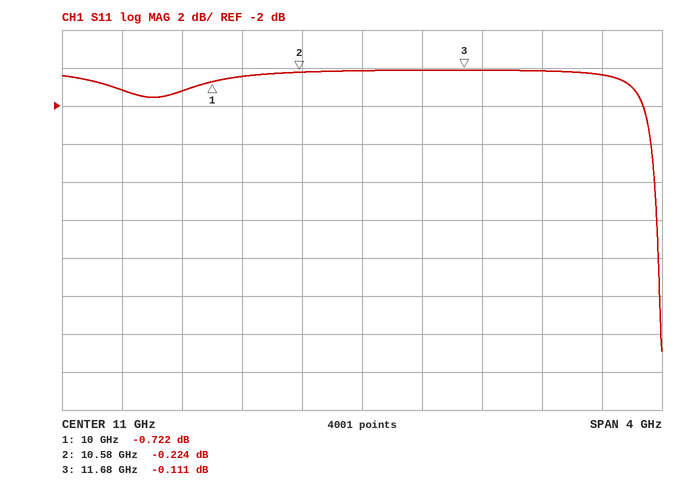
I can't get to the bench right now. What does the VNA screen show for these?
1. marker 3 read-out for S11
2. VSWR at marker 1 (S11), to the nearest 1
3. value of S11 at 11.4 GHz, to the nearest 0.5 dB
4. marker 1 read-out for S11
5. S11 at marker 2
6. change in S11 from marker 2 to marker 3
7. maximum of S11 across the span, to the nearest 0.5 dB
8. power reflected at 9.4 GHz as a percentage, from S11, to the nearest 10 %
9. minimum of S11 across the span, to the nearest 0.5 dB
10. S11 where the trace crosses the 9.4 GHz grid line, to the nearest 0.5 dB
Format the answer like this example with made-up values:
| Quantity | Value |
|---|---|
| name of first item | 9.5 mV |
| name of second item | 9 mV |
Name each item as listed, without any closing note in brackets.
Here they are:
| Quantity | Value |
|---|---|
| marker 3 read-out for S11 | -0.111 dB |
| VSWR at marker 1 (S11), to the nearest 1 | 24 |
| value of S11 at 11.4 GHz, to the nearest 0.5 dB | 0.0 dB |
| marker 1 read-out for S11 | -0.722 dB |
| S11 at marker 2 | -0.224 dB |
| change in S11 from marker 2 to marker 3 | 0.113 dB |
| maximum of S11 across the span, to the nearest 0.5 dB | 0.0 dB |
| power reflected at 9.4 GHz as a percentage, from S11, to the nearest 10 % | 80 % |
| minimum of S11 across the span, to the nearest 0.5 dB | -15.0 dB |
| S11 where the trace crosses the 9.4 GHz grid line, to the nearest 0.5 dB | -1.0 dB |
